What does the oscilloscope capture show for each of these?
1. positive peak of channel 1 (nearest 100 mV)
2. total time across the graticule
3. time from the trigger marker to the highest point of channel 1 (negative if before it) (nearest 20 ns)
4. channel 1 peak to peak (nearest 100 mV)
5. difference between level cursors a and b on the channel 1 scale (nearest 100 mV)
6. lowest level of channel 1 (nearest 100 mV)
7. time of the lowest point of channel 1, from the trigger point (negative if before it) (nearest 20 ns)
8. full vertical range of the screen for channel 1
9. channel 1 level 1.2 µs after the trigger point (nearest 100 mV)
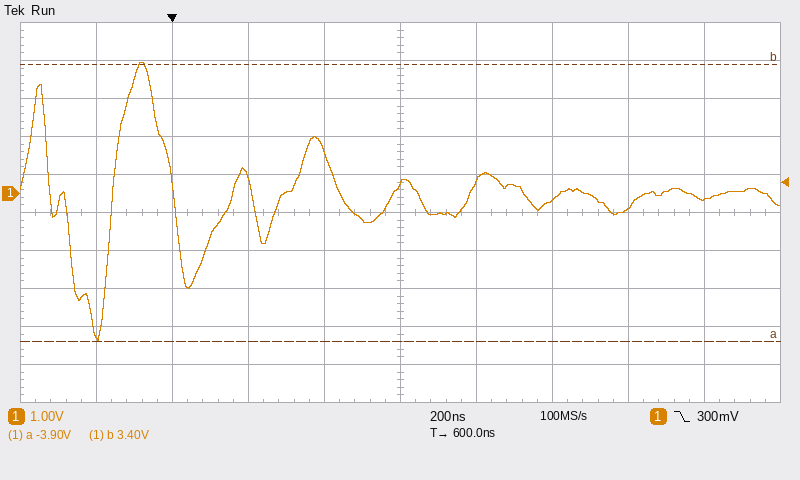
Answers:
3.4 V
2 µs
-80 ns
7.3 V
7.3 V
-3.9 V
-200 ns
10 V
-400 mV
